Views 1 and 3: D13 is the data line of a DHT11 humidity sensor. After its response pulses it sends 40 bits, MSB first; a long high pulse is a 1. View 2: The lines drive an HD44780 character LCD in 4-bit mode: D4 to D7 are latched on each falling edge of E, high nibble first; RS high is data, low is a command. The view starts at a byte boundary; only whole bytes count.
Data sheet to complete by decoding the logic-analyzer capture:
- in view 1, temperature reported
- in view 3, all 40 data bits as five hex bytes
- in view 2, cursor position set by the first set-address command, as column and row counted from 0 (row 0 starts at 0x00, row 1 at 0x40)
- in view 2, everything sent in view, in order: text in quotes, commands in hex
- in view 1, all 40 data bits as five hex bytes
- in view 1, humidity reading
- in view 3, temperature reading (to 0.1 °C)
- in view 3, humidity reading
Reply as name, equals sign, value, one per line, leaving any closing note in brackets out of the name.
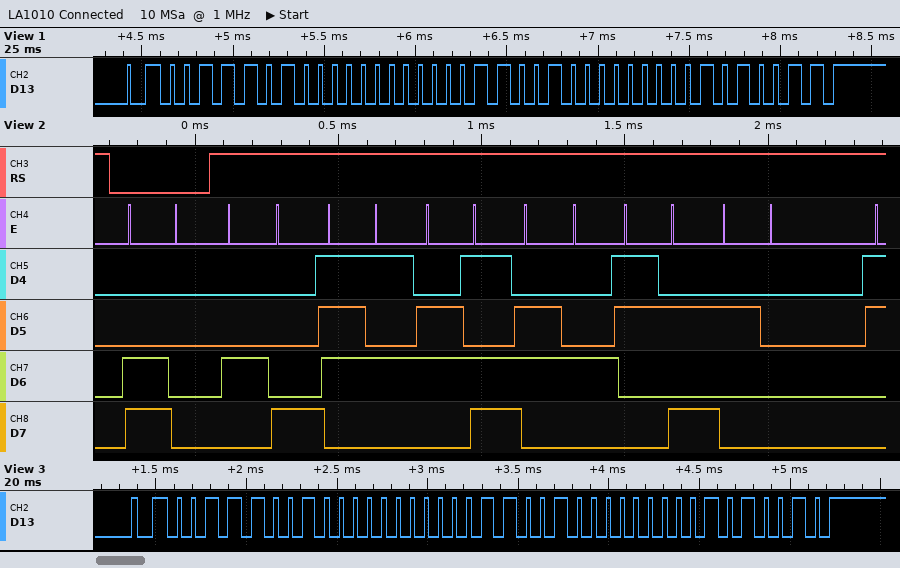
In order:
in view 1, temperature reported = 25.0 °C
in view 3, all 40 data bits as five hex bytes = 39 00 19 00 52
in view 2, cursor position set by the first set-address command, as column and row counted from 0 = column 0, row 1
in view 2, everything sent in view, in order: text in quotes, commands in hex = 0xC0 "Humd: "
in view 1, all 40 data bits as five hex bytes = 3A 00 19 00 53
in view 1, humidity reading = 58 %
in view 3, temperature reading = 25.0 °C
in view 3, humidity reading = 57 %
